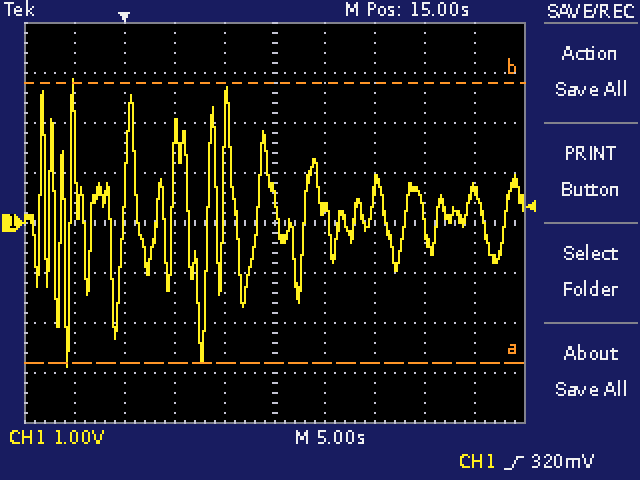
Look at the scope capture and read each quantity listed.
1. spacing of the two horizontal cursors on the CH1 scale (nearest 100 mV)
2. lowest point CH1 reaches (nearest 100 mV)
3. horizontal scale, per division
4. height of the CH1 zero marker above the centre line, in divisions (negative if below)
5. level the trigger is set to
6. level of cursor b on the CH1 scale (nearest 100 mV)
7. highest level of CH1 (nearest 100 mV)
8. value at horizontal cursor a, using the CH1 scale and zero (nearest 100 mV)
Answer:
5.6 V
-2.9 V
5 s
0.0 div
320 mV
2.8 V
2.9 V
-2.8 V
